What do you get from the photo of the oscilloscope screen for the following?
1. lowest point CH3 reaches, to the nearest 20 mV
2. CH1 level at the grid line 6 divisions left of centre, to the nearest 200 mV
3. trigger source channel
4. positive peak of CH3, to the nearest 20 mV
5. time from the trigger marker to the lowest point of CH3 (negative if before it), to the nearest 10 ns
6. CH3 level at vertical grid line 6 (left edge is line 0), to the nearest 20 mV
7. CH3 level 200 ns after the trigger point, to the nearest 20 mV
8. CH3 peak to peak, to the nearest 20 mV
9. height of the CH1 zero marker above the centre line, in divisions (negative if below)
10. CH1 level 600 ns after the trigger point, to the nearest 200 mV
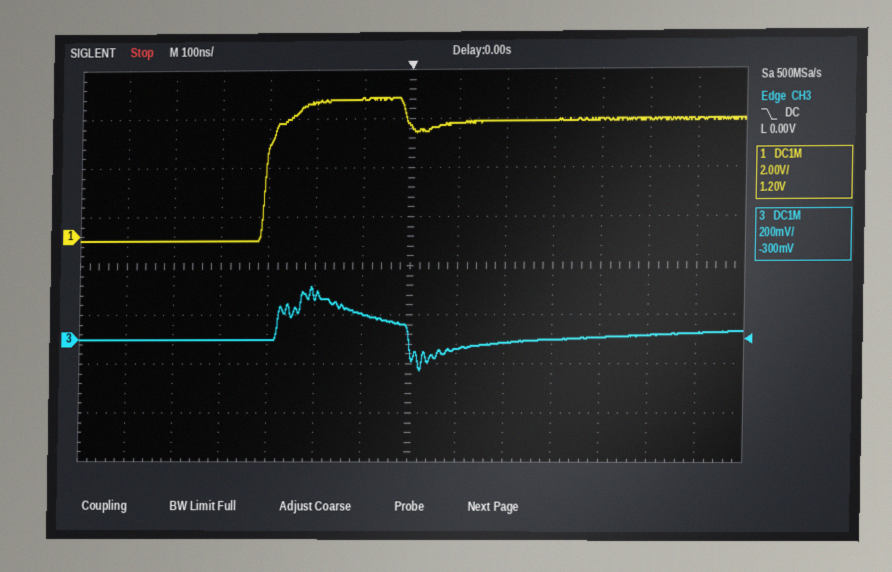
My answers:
-120 mV
-200 mV
CH3
220 mV
+20 ns
100 mV
-20 mV
340 mV
+0.6 div
4.8 V
